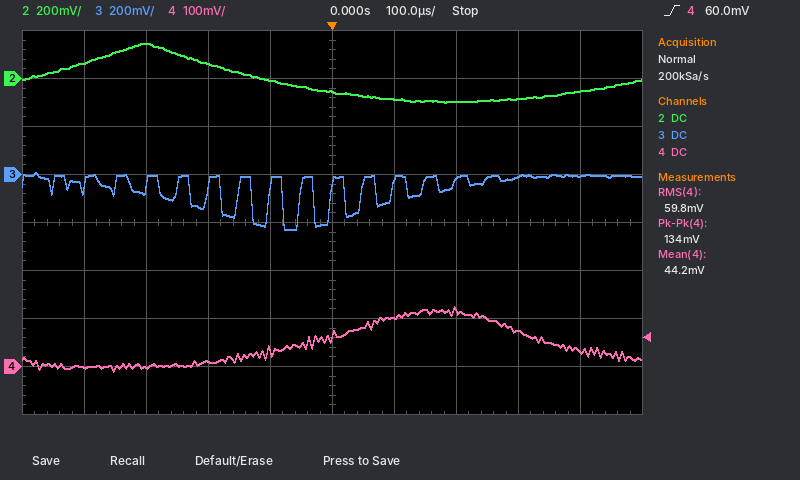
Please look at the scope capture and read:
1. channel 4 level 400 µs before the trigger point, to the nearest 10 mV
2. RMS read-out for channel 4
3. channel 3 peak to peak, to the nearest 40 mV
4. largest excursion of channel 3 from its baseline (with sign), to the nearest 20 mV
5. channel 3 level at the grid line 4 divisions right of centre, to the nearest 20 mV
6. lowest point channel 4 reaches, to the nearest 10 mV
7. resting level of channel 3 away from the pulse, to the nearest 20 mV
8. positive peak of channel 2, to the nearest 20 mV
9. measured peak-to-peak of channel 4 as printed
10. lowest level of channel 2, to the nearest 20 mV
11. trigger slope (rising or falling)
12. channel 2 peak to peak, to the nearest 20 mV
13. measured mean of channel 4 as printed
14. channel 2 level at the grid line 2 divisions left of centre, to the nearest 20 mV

0 mV
59.8 mV
240 mV
-220 mV
0 mV
-10 mV
0 mV
140 mV
134 mV
-100 mV
rising
240 mV
44.2 mV
60 mV
